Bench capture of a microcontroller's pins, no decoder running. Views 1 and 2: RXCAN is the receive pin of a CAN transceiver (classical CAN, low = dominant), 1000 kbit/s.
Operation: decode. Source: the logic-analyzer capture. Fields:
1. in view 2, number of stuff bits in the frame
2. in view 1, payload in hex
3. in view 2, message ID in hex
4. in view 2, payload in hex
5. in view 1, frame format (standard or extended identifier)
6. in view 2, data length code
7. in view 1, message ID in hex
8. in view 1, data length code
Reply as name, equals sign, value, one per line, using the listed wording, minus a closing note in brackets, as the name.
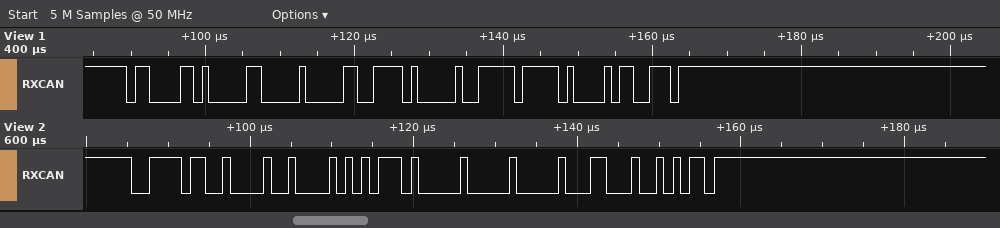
in view 2, number of stuff bits in the frame = 3
in view 1, payload in hex = 00 9E 80 FF
in view 2, message ID in hex = 0x3D9
in view 2, payload in hex = 85 5D 00 00
in view 1, frame format = standard
in view 2, data length code = 4
in view 1, message ID in hex = 0x61A
in view 1, data length code = 4
